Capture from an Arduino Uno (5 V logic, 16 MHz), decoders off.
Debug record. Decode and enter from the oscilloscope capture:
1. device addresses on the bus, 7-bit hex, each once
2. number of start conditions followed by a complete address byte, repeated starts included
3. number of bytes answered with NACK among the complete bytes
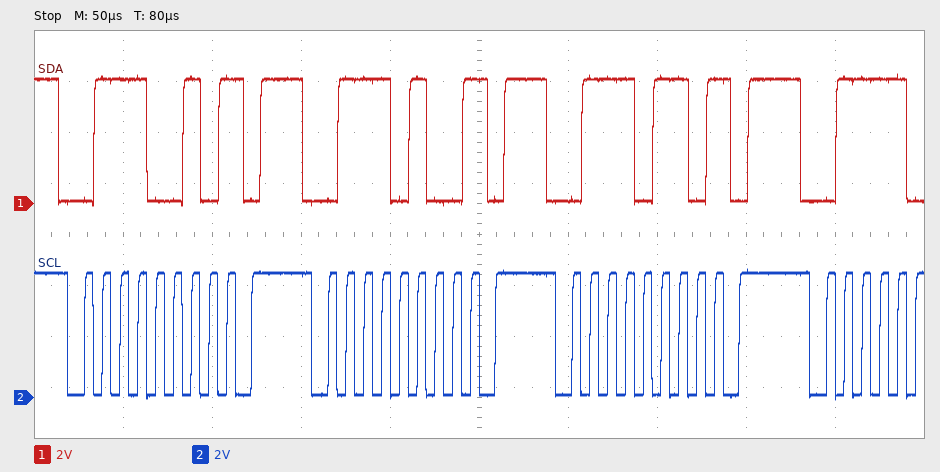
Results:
0x39 0x3A 0x3B
3
3
